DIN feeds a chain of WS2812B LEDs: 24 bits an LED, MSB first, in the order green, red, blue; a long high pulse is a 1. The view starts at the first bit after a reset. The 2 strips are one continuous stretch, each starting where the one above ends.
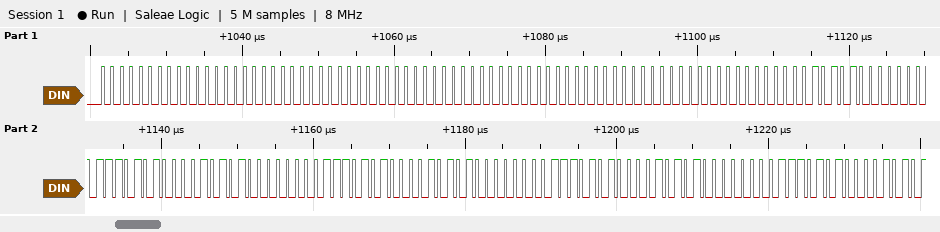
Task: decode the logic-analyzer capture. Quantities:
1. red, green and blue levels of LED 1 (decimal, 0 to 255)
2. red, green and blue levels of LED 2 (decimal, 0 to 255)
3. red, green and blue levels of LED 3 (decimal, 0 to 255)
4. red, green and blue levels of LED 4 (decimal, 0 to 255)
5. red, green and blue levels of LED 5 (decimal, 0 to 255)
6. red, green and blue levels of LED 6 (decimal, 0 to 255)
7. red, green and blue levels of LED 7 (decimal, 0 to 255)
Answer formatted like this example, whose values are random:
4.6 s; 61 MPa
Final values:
0, 0, 0; 0, 0, 0; 0, 0, 0; 0, 21, 234; 0, 21, 234; 0, 21, 234; 0, 21, 234
